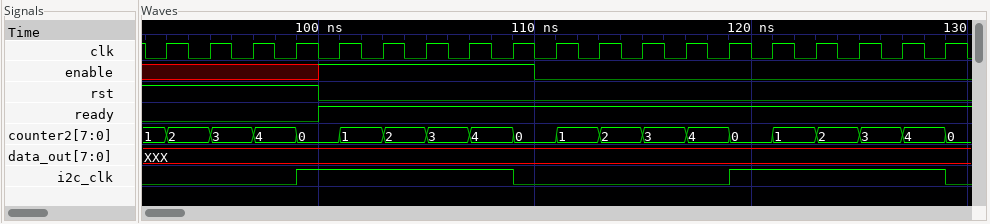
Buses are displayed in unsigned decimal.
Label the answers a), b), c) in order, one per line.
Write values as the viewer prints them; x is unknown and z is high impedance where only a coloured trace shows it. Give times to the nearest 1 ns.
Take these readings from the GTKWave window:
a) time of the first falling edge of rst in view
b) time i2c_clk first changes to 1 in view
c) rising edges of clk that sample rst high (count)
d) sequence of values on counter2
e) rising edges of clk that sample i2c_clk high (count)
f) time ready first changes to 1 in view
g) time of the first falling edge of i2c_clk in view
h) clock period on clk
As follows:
a) 100 ns
b) 99 ns
c) 4
d) 1, 2, 3, 4, 0, 1, 2, 3, 4, 0, 1, 2, 3, 4, 0, 1, 2, 3, 4, 0
e) 10
f) 100 ns
g) 109 ns
h) 2 ns
